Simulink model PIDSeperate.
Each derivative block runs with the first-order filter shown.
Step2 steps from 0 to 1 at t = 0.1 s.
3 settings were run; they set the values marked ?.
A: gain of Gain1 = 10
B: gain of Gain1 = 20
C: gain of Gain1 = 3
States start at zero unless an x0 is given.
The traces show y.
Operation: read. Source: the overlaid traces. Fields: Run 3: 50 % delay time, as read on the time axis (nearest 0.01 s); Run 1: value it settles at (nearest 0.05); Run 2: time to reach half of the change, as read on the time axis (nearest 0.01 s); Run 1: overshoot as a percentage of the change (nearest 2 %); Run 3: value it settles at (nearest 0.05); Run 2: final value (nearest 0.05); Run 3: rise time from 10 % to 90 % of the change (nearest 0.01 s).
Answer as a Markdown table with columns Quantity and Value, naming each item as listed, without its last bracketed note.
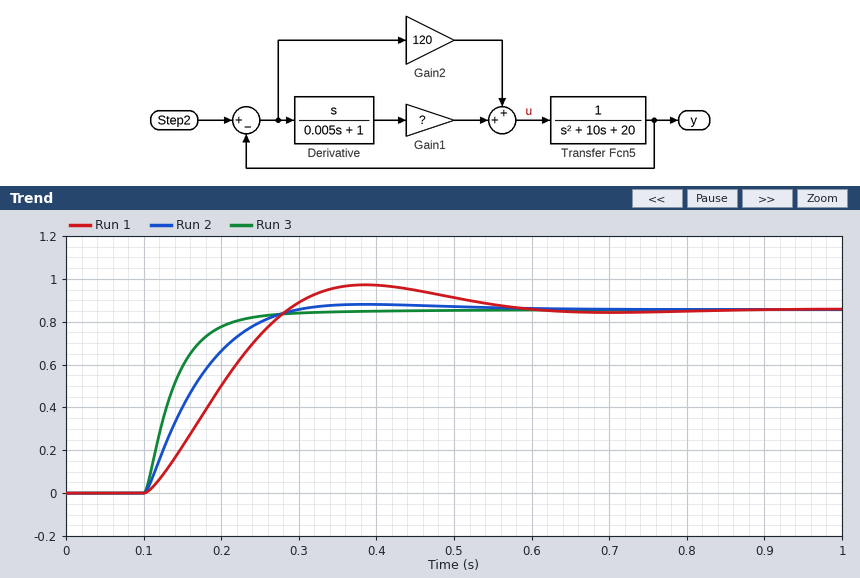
| Quantity | Value |
|---|---|
| Run 3: 50 % delay time, as read on the time axis | 0.13 s |
| Run 1: value it settles at | 0.85 |
| Run 2: time to reach half of the change, as read on the time axis | 0.15 s |
| Run 1: overshoot as a percentage of the change | 14 % |
| Run 3: value it settles at | 0.85 |
| Run 2: final value | 0.85 |
| Run 3: rise time from 10 % to 90 % of the change | 0.09 s |
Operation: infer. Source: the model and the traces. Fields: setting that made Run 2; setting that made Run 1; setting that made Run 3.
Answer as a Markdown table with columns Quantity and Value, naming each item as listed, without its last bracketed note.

| Quantity | Value |
|---|---|
| setting that made Run 2 | A |
| setting that made Run 1 | C |
| setting that made Run 3 | B |
